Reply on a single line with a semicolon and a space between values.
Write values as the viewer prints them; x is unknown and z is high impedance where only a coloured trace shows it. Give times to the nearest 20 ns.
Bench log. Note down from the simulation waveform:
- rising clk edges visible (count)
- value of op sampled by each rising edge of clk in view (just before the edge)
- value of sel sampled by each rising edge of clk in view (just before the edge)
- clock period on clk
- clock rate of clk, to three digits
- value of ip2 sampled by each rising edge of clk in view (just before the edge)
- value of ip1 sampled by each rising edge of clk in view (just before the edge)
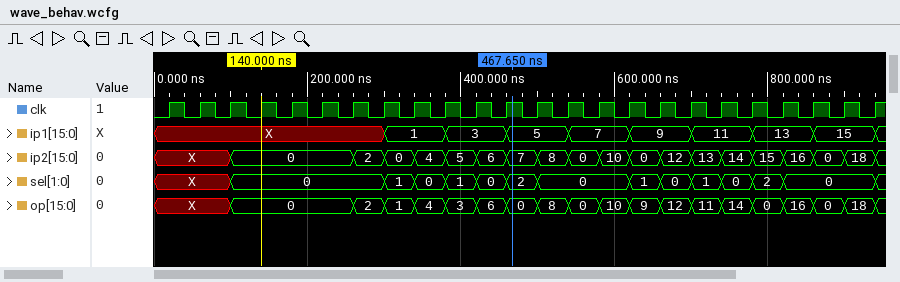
24; X, X, X, 0, 0, 0, 0, 2, 1, 4, 3, 6, 0, 8, 0, 10, 9, 12, 11, 14, 0, 16, 0, 18; X, X, X, 0, 0, 0, 0, 0, 1, 0, 1, 0, 2, 0, 0, 0, 1, 0, 1, 0, 2, 0, 0, 0; 40 ns; 25.0 MHz; X, X, X, 0, 0, 0, 0, 2, 0, 4, 5, 6, 7, 8, 0, 10, 0, 12, 13, 14, 15, 16, 0, 18; X, X, X, X, X, X, X, X, 1, 1, 3, 3, 5, 5, 7, 7, 9, 9, 11, 11, 13, 13, 15, 15
